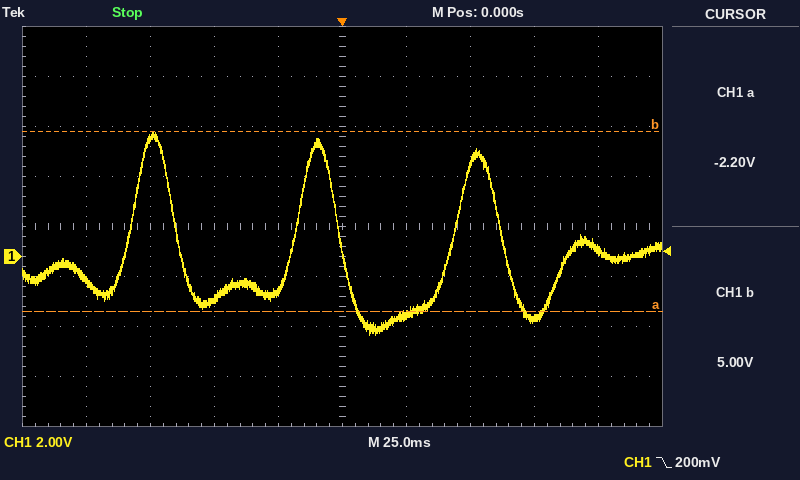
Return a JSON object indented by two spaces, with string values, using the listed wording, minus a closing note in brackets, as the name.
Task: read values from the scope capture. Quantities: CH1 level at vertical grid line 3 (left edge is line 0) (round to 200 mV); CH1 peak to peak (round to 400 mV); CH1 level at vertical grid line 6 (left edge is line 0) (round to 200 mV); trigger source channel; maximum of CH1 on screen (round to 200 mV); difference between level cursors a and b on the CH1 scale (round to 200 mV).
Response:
{
  "CH1 level at vertical grid line 3 (left edge is line 0)": "-1.6 V",
  "CH1 peak to peak": "8.0 V",
  "CH1 level at vertical grid line 6 (left edge is line 0)": "-2.4 V",
  "trigger source channel": "CH1",
  "maximum of CH1 on screen": "5.0 V",
  "difference between level cursors a and b on the CH1 scale": "7.2 V"
}
